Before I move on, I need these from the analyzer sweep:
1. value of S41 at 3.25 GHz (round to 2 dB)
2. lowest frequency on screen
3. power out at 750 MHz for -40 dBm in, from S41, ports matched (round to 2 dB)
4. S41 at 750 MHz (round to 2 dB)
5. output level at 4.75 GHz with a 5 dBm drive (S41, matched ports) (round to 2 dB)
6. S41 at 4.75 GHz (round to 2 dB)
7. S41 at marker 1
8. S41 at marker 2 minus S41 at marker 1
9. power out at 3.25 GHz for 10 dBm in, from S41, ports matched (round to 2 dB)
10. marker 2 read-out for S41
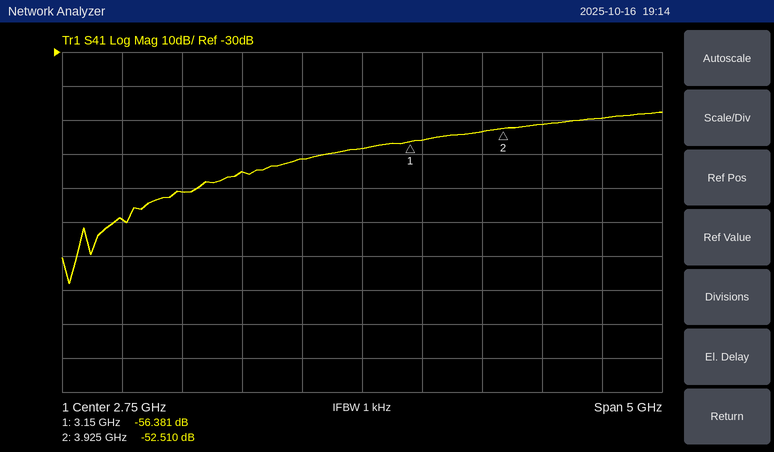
-56 dB
250 MHz
-120 dBm
-80 dB
-44 dBm
-50 dB
-56.381 dB
3.871 dB
-46 dBm
-52.510 dB
